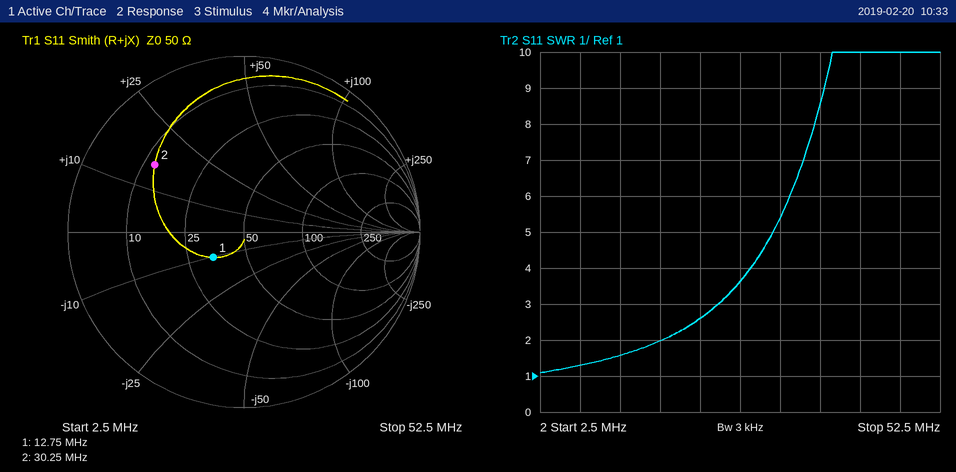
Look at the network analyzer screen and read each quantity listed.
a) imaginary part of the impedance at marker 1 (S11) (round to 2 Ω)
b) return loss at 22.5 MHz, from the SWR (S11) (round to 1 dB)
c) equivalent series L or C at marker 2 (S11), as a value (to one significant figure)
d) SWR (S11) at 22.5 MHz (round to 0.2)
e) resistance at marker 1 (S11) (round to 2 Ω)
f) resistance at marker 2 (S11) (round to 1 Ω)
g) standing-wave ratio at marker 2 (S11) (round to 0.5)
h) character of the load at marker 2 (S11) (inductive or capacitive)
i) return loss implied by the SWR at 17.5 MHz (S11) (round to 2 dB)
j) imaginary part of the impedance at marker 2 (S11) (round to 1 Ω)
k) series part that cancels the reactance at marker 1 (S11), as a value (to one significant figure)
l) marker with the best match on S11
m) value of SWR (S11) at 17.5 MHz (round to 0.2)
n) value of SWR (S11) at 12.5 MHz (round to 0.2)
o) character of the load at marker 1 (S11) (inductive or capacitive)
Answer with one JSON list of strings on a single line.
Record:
["-10 Ω", "7 dB", "80 nH", "2.6", "34 Ω", "12 Ω", "4.5", "inductive", "10 dB", "+16 Ω", "100 nH", "marker 1", "2.0", "1.6", "capacitive"]
